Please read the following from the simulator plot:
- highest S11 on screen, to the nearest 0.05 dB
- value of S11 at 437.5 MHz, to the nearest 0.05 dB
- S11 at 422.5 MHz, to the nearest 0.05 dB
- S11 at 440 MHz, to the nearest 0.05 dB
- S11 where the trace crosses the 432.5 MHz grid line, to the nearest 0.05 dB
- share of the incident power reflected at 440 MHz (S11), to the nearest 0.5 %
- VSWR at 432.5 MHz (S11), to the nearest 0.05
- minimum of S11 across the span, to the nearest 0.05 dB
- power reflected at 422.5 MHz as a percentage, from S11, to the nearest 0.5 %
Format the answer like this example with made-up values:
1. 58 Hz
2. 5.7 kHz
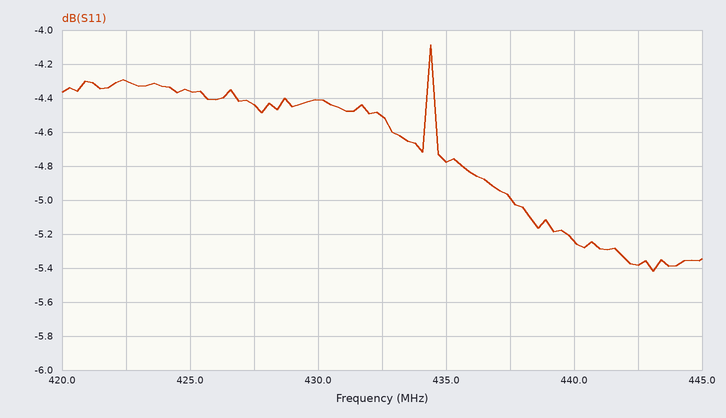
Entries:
1. -4.10 dB
2. -5.00 dB
3. -4.30 dB
4. -5.25 dB
5. -4.50 dB
6. 30.0 %
7. 3.95
8. -5.40 dB
9. 37.0 %
